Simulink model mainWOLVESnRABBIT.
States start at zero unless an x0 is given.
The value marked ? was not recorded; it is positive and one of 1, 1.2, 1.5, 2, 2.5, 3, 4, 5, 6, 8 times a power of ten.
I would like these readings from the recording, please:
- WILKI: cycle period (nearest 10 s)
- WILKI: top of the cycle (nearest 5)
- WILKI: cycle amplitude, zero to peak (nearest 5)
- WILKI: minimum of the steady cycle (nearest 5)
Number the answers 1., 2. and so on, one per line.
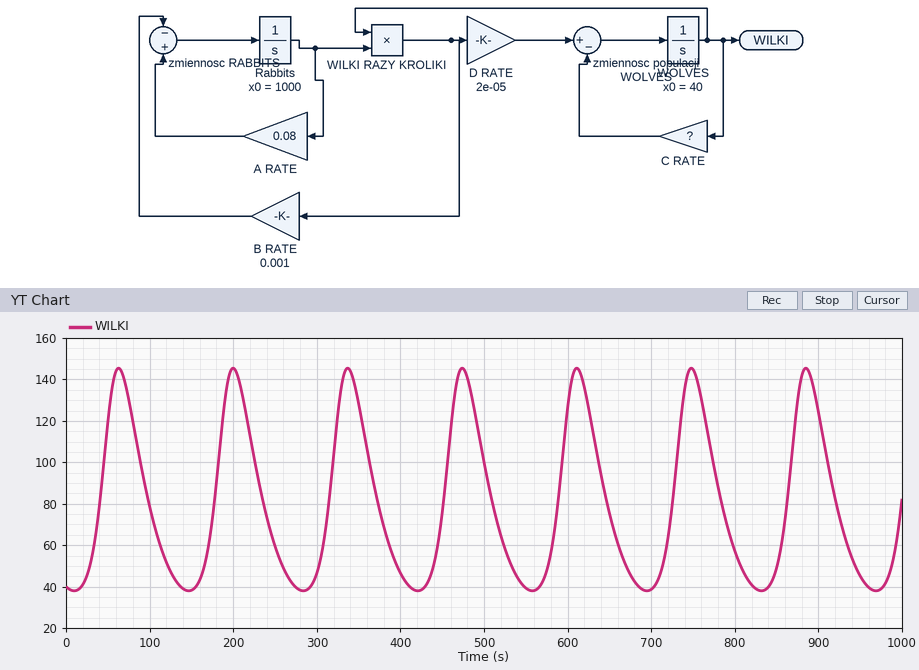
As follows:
1. 140 s
2. 145
3. 55
4. 40
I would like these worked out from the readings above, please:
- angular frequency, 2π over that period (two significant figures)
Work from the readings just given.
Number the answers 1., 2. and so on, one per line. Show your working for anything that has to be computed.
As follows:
1. 2π / 140 = 0.045 rad/s
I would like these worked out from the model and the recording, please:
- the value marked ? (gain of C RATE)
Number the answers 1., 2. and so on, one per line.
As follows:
1. 0.03
